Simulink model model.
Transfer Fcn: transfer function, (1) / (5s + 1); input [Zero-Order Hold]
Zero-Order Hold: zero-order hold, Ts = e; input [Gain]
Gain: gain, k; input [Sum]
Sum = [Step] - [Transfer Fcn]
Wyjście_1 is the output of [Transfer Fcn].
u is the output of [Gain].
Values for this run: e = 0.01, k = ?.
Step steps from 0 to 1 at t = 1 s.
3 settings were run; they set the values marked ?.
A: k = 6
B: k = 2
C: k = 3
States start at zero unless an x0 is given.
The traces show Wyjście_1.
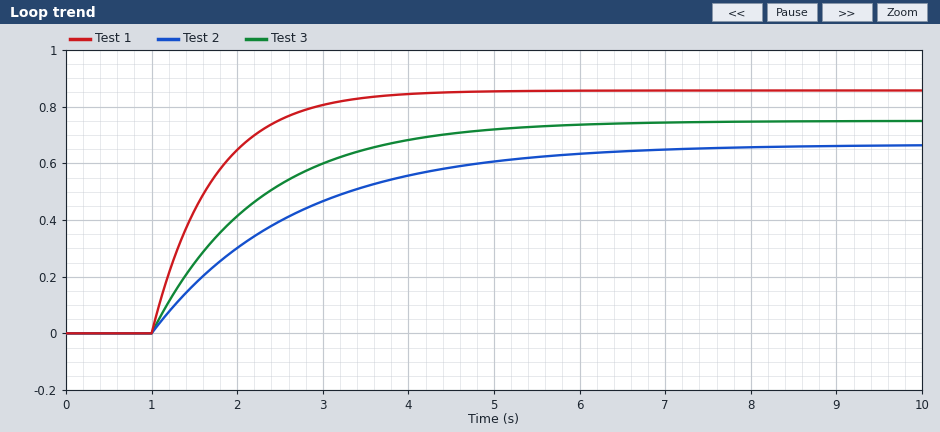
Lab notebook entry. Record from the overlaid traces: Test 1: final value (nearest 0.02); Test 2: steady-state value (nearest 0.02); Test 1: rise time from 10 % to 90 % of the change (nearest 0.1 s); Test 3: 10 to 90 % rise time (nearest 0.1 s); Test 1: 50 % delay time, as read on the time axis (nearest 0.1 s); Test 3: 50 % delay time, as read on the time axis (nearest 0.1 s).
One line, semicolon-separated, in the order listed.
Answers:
0.86; 0.66; 1.6 s; 2.7 s; 1.5 s; 1.9 s
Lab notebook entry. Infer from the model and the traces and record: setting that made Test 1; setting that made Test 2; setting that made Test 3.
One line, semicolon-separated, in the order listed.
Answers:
A; B; C
